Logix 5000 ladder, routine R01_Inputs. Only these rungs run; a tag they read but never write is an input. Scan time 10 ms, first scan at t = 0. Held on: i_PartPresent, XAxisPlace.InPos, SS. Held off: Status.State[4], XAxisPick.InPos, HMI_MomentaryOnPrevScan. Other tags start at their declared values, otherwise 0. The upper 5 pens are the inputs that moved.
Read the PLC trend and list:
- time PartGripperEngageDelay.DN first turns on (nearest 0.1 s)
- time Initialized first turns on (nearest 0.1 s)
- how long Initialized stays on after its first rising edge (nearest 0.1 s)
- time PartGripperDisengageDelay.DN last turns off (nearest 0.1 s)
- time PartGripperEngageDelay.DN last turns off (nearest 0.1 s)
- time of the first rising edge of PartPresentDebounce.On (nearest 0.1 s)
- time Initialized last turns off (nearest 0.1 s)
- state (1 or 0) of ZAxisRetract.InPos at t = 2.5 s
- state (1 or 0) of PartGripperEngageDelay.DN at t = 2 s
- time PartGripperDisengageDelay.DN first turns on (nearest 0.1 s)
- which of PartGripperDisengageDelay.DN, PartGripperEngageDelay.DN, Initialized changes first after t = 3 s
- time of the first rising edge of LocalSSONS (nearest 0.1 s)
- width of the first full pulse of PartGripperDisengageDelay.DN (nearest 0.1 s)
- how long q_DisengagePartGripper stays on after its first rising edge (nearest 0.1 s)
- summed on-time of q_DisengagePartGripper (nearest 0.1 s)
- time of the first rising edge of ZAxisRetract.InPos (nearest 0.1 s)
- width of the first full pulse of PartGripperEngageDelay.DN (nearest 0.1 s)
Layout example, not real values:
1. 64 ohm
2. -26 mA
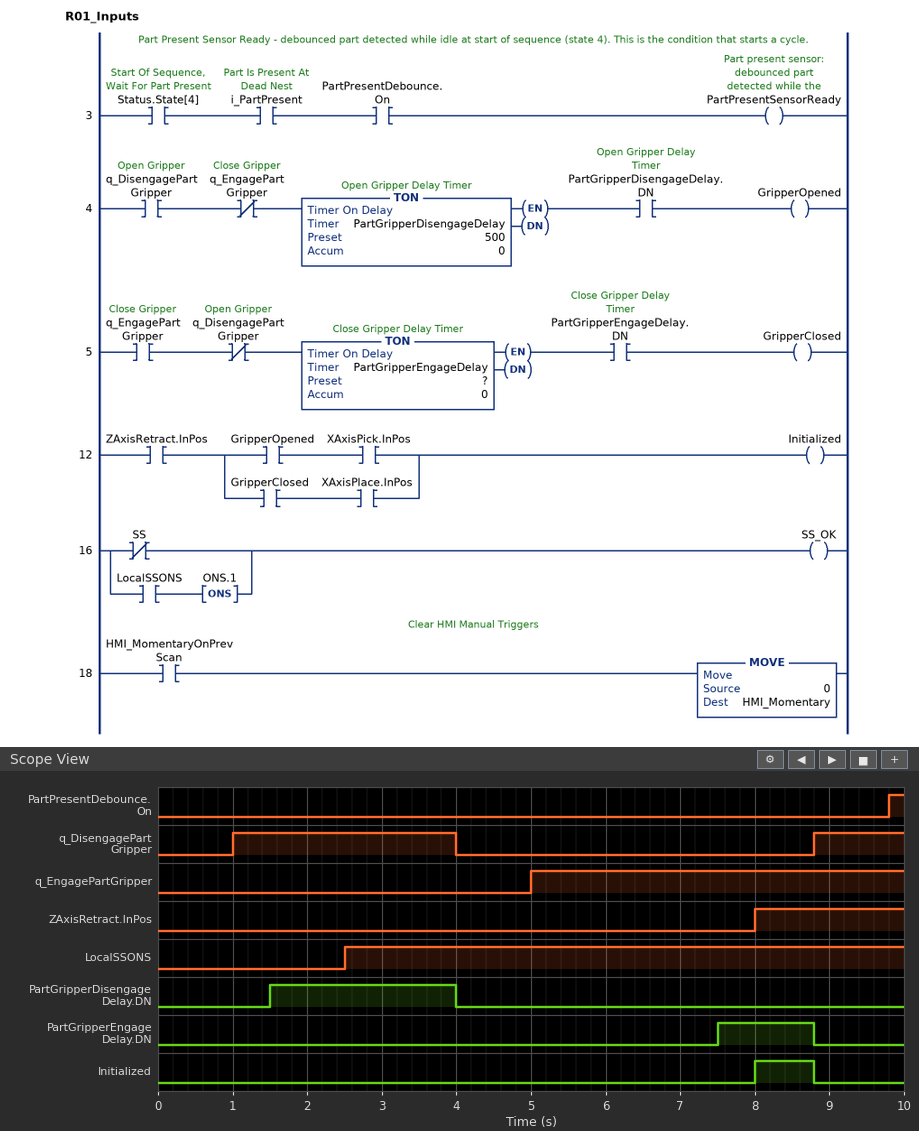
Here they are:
1. 7.5 s
2. 8.0 s
3. 0.8 s
4. 4.0 s
5. 8.8 s
6. 9.8 s
7. 8.8 s
8. 0
9. 0
10. 1.5 s
11. PartGripperDisengageDelay.DN
12. 2.5 s
13. 2.5 s
14. 3.0 s
15. 4.2 s
16. 8.0 s
17. 1.3 s
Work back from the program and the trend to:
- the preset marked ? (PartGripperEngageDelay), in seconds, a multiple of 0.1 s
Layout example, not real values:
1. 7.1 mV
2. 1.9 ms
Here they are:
1. 2.5 s
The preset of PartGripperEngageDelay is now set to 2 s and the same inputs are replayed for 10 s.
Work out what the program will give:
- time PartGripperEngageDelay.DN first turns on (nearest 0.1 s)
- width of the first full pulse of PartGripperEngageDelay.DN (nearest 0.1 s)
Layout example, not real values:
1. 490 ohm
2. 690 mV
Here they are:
1. 7.0 s
2. 1.8 s
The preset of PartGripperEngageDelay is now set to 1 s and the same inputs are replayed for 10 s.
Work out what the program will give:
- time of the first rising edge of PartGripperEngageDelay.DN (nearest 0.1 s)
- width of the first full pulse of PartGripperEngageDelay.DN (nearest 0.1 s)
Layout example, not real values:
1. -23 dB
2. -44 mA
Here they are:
1. 6.0 s
2. 2.8 s
